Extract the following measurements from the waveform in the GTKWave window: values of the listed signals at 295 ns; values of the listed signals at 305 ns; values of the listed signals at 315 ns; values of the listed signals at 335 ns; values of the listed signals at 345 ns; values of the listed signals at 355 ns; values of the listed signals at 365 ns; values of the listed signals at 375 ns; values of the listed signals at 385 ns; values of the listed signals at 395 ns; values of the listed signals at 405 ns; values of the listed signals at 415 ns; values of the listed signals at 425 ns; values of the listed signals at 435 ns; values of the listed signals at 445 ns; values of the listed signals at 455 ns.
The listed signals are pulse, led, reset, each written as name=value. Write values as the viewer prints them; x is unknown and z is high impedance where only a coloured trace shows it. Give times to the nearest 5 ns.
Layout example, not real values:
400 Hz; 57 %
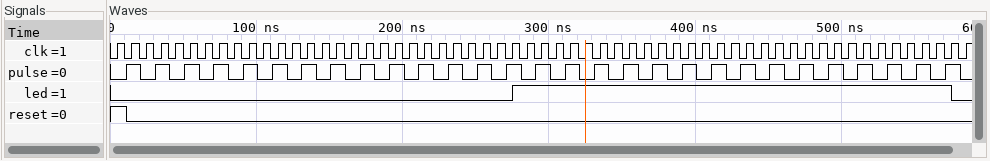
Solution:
pulse=1, led=1, reset=0; pulse=0, led=1, reset=0; pulse=1, led=1, reset=0; pulse=1, led=1, reset=0; pulse=0, led=1, reset=0; pulse=1, led=1, reset=0; pulse=0, led=1, reset=0; pulse=1, led=1, reset=0; pulse=0, led=1, reset=0; pulse=1, led=1, reset=0; pulse=0, led=1, reset=0; pulse=1, led=1, reset=0; pulse=0, led=1, reset=0; pulse=1, led=1, reset=0; pulse=0, led=1, reset=0; pulse=1, led=1, reset=0
